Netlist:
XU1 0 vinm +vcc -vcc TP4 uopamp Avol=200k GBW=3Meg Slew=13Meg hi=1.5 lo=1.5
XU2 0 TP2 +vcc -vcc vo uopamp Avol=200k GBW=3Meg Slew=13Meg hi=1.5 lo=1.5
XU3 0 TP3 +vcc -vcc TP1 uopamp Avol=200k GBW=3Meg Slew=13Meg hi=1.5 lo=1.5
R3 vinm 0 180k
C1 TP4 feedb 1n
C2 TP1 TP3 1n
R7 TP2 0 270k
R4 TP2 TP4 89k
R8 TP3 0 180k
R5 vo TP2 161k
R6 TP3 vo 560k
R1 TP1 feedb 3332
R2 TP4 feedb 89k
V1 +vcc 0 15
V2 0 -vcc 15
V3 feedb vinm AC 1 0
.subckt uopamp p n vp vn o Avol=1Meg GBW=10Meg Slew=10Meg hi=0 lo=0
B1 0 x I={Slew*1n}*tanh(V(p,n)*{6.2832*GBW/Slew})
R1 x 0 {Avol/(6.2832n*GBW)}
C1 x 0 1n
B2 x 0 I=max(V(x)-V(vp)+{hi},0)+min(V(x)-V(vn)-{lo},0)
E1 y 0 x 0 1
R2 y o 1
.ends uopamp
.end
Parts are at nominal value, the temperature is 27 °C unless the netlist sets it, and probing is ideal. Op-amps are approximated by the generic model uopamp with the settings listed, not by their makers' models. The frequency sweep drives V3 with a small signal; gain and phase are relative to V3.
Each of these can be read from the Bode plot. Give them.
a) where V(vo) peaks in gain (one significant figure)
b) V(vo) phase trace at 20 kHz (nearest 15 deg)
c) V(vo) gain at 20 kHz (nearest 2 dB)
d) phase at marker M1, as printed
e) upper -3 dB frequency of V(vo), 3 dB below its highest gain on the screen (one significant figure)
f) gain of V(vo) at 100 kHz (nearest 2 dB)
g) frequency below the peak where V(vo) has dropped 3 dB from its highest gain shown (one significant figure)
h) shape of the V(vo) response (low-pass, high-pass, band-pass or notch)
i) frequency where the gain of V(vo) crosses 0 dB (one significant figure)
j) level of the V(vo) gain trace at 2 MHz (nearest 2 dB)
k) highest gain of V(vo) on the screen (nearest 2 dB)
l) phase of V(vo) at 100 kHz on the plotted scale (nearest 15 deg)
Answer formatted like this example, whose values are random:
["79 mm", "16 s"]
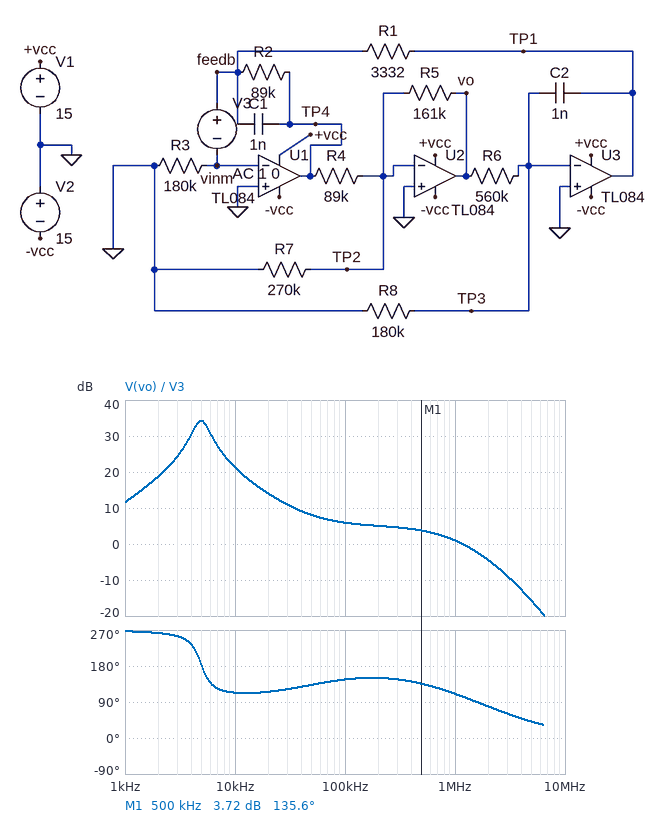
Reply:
["5 kHz", "120 deg", "14 dB", "135.6 deg", "6 kHz", "6 dB", "4 kHz", "band-pass", "1 MHz", "-4 dB", "34 dB", "150 deg"]
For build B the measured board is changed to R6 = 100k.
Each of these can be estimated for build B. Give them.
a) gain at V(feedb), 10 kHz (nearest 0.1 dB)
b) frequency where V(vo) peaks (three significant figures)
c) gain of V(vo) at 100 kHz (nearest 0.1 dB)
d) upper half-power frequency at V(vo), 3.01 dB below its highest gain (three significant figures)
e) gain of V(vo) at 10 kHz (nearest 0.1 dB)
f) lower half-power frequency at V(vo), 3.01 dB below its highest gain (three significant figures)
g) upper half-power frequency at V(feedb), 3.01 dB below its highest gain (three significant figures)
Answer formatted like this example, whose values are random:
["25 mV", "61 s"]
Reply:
["0.4 dB", "11.6 kHz", "6.0 dB", "12.4 kHz", "27.4 dB", "10.9 kHz", "2.50 MHz"]
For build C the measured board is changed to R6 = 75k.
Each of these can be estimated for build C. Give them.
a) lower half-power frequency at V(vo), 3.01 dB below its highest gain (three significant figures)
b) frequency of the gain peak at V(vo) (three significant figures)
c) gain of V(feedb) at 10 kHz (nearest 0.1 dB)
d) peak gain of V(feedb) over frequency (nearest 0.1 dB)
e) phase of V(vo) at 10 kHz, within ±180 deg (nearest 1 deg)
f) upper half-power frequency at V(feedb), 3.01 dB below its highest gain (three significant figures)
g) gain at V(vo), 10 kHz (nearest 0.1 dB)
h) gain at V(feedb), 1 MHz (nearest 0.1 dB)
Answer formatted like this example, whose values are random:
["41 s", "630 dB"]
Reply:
["12.7 kHz", "13.4 kHz", "0.2 dB", "0.8 dB", "-90 deg", "2.38 MHz", "20.9 dB", "-0.6 dB"]
